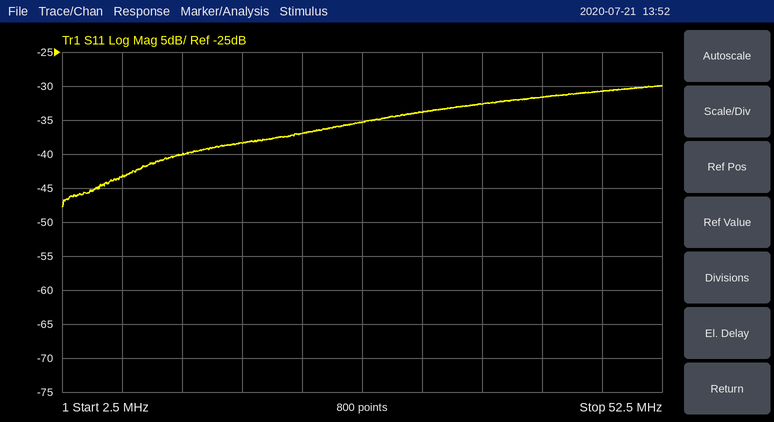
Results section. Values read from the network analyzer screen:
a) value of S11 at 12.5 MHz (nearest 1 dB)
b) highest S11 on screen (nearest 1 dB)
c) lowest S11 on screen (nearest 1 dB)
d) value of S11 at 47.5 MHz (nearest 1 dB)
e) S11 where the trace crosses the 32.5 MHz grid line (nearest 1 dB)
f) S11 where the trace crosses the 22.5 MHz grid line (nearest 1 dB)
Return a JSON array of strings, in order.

["-40 dB", "-30 dB", "-48 dB", "-31 dB", "-34 dB", "-37 dB"]
